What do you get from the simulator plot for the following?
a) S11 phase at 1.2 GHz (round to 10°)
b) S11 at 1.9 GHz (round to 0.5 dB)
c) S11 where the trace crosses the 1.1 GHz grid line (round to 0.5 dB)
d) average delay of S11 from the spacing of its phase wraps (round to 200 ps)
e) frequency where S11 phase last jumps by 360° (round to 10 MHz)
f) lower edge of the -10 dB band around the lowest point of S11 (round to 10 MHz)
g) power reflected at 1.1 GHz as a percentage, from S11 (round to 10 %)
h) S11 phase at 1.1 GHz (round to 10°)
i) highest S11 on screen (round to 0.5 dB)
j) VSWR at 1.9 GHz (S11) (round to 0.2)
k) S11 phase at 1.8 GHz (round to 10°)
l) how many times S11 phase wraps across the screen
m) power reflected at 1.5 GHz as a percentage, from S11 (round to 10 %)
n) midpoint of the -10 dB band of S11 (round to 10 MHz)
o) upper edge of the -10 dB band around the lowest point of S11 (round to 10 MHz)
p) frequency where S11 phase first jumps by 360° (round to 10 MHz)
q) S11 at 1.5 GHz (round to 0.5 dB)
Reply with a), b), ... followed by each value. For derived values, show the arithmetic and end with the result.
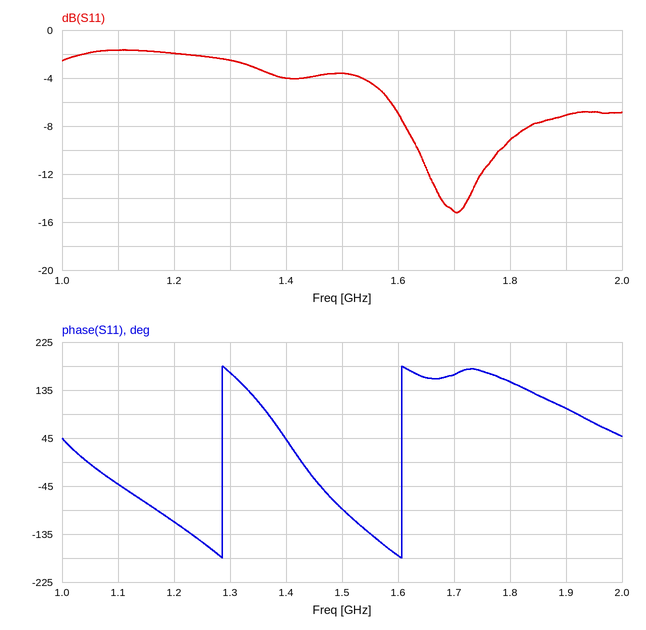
a) -110°
b) -7.0 dB
c) -1.5 dB
d) 1 cycle / (1.61 GHz − 1.29 GHz) ≈ 3.12 ns, so 3.2 ns to the nearest 200 ps
e) 1.61 GHz
f) 1.64 GHz
g) 10^(-1.5/10) ≈ 70.8 %, so 70 % to the nearest 10 %
h) -40°
i) -1.5 dB
j) |Γ| = 10^(-7/20) = 0.4467; VSWR = (1 + 0.4467)/(1 − 0.4467) ≈ 2.6
k) 150°
l) 2
m) 10^(-3.5/10) ≈ 44.7 %, so 40 % to the nearest 10 %
n) 1.71 GHz
o) 1.78 GHz
p) 1.29 GHz
q) -3.5 dB
